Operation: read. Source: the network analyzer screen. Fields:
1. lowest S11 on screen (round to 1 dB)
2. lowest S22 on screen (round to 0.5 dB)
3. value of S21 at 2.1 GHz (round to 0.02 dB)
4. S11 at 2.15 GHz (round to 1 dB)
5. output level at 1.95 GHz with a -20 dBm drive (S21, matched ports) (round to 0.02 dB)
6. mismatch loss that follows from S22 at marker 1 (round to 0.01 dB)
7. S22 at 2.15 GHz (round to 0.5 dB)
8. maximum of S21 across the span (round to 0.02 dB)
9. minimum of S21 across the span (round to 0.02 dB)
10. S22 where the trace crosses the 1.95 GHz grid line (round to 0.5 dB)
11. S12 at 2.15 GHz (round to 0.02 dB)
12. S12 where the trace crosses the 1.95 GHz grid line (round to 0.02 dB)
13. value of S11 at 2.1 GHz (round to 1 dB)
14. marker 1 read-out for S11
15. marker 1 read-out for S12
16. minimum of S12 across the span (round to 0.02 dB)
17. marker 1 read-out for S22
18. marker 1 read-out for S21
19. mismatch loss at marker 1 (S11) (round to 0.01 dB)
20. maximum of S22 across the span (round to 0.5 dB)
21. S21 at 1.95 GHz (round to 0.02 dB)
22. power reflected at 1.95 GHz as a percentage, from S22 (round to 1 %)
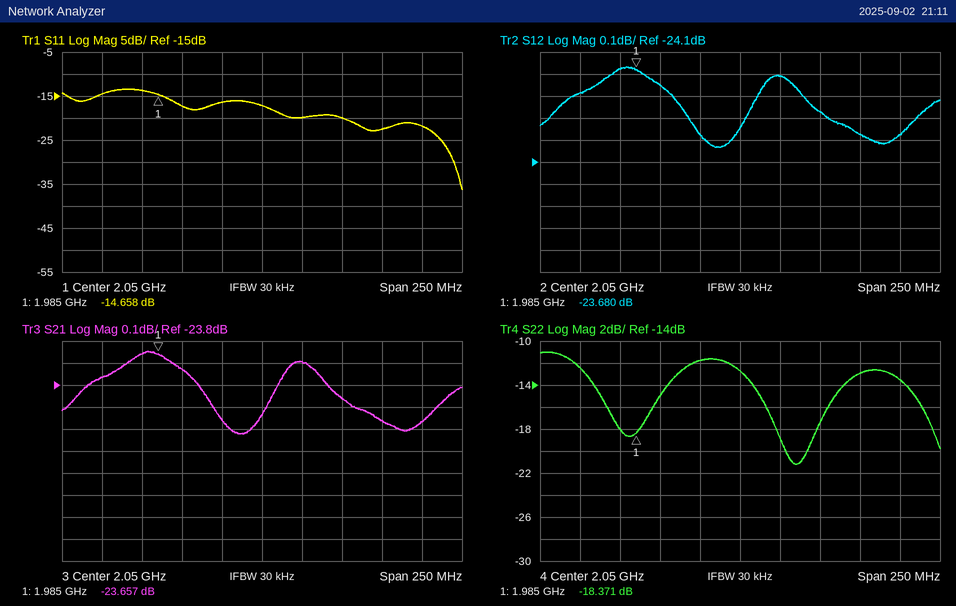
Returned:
-36 dB
-21.0 dB
-23.86 dB
-22 dB
-43.76 dBm
0.06 dB
-13.5 dB
-23.64 dB
-24.02 dB
-12.5 dB
-23.98 dB
-23.78 dB
-20 dB
-14.658 dB
-23.680 dB
-24.04 dB
-18.371 dB
-23.657 dB
0.15 dB
-11.0 dB
-23.76 dB
6 %
